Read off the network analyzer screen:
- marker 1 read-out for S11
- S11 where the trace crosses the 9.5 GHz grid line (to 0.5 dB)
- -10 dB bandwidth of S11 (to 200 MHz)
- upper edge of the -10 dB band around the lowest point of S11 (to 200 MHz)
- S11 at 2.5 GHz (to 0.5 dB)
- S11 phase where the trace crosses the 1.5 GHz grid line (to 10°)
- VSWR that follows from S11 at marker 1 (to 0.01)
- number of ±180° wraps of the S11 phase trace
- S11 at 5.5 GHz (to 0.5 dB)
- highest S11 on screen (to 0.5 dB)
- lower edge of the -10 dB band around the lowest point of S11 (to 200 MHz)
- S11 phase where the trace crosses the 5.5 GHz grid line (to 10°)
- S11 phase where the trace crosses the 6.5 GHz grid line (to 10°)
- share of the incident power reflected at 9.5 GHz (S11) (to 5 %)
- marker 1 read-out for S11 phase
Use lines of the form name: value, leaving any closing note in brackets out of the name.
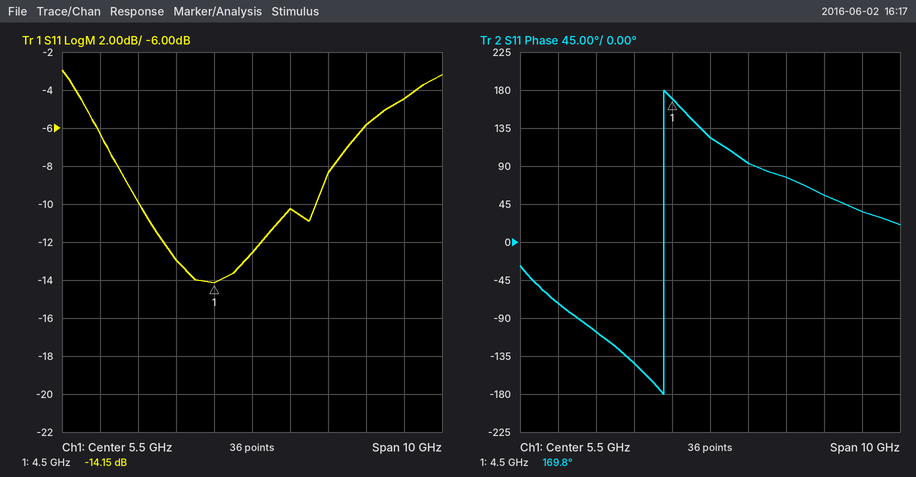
marker 1 read-out for S11: -14.15 dB
S11 where the trace crosses the 9.5 GHz grid line: -4.5 dB
-10 dB bandwidth of S11: 4.6 GHz
upper edge of the -10 dB band around the lowest point of S11: 7.2 GHz
S11 at 2.5 GHz: -10.0 dB
S11 phase where the trace crosses the 1.5 GHz grid line: -70°
VSWR that follows from S11 at marker 1: 1.49
number of ±180° wraps of the S11 phase trace: 1
S11 at 5.5 GHz: -12.5 dB
highest S11 on screen: -3.0 dB
lower edge of the -10 dB band around the lowest point of S11: 2.6 GHz
S11 phase where the trace crosses the 5.5 GHz grid line: 120°
S11 phase where the trace crosses the 6.5 GHz grid line: 90°
share of the incident power reflected at 9.5 GHz (S11): 35 %
marker 1 read-out for S11 phase: 169.8°
